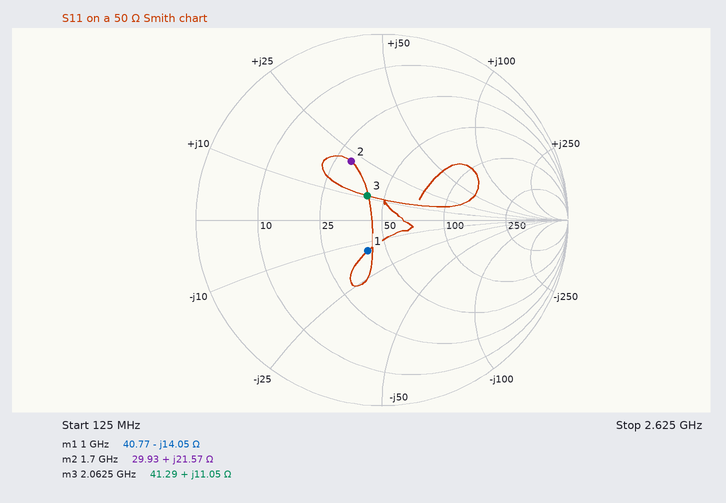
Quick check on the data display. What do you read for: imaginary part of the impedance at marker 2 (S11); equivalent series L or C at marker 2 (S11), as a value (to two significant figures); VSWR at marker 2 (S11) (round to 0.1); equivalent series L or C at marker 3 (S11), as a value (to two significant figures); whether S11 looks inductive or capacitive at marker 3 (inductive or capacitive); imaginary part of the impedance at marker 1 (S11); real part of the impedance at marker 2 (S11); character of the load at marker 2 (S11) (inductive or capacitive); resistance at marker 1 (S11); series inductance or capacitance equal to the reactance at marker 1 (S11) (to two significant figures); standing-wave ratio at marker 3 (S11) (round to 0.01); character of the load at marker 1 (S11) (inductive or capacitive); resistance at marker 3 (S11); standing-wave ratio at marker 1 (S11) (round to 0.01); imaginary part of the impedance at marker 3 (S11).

+21.57 Ω
2.0 nH
2.1
850 pH
inductive
-14.05 Ω
29.93 Ω
inductive
40.77 Ω
11 pF
1.36
capacitive
41.29 Ω
1.45
+11.05 Ω
